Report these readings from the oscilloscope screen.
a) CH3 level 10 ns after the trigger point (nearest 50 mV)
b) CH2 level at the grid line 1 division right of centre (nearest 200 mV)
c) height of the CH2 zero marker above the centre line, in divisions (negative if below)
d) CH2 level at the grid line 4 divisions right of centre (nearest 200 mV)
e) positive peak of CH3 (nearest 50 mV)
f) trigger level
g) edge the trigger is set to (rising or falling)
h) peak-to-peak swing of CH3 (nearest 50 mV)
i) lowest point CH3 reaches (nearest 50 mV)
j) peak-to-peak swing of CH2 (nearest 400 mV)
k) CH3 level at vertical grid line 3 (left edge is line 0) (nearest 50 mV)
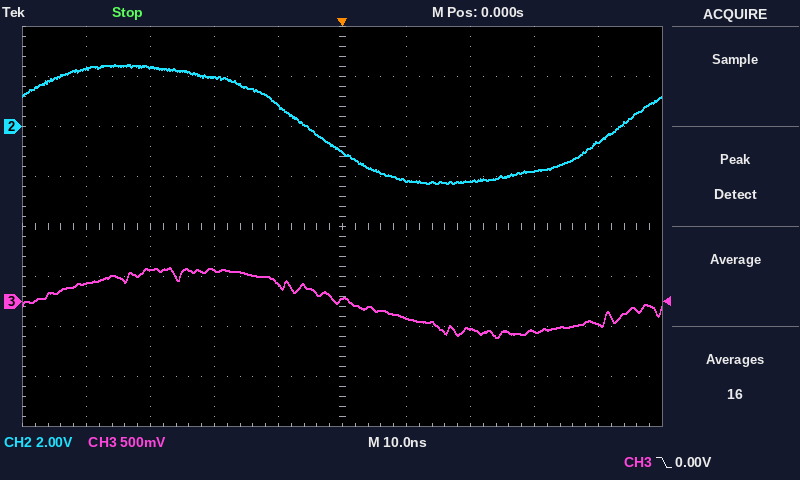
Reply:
-150 mV
-2.2 V
+2.0 div
-600 mV
350 mV
0.00 V
falling
700 mV
-350 mV
4.8 V
300 mV
